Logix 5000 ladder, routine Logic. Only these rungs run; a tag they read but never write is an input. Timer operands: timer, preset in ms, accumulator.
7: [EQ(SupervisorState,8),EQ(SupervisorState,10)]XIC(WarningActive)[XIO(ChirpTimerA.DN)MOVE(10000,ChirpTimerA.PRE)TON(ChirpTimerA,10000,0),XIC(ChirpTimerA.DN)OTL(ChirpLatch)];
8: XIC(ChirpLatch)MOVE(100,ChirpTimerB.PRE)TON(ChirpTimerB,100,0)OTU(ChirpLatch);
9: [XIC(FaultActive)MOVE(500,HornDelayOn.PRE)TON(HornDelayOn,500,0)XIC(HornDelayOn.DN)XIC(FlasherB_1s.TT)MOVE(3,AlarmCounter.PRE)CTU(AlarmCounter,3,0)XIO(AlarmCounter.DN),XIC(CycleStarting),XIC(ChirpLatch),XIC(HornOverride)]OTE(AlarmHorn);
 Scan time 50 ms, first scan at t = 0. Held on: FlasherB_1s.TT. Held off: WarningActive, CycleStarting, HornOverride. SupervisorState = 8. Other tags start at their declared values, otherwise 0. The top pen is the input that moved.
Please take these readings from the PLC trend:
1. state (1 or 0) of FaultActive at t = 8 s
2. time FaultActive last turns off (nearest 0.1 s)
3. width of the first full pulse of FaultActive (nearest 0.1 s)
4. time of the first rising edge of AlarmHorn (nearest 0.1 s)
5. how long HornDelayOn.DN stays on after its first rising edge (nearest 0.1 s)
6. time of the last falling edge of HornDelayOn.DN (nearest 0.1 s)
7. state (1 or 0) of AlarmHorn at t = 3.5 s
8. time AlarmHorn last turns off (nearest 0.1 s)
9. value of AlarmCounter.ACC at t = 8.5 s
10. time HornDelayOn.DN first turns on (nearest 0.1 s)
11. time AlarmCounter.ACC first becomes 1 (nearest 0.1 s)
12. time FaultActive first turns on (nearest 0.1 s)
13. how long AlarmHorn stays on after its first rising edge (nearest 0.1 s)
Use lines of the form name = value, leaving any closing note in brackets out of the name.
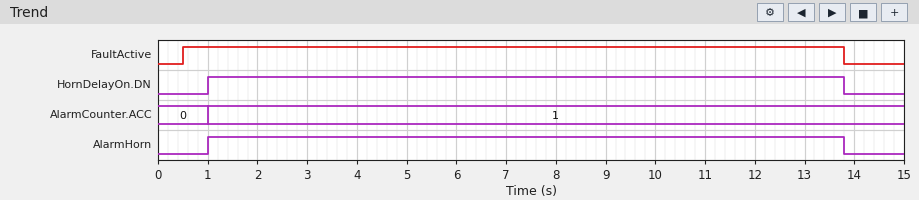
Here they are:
state (1 or 0) of FaultActive at t = 8 s = 1
time FaultActive last turns off = 13.8 s
width of the first full pulse of FaultActive = 13.3 s
time of the first rising edge of AlarmHorn = 1.0 s
how long HornDelayOn.DN stays on after its first rising edge = 12.8 s
time of the last falling edge of HornDelayOn.DN = 13.8 s
state (1 or 0) of AlarmHorn at t = 3.5 s = 1
time AlarmHorn last turns off = 13.8 s
value of AlarmCounter.ACC at t = 8.5 s = 1
time HornDelayOn.DN first turns on = 1.0 s
time AlarmCounter.ACC first becomes 1 = 1.0 s
time FaultActive first turns on = 0.5 s
how long AlarmHorn stays on after its first rising edge = 12.8 s
